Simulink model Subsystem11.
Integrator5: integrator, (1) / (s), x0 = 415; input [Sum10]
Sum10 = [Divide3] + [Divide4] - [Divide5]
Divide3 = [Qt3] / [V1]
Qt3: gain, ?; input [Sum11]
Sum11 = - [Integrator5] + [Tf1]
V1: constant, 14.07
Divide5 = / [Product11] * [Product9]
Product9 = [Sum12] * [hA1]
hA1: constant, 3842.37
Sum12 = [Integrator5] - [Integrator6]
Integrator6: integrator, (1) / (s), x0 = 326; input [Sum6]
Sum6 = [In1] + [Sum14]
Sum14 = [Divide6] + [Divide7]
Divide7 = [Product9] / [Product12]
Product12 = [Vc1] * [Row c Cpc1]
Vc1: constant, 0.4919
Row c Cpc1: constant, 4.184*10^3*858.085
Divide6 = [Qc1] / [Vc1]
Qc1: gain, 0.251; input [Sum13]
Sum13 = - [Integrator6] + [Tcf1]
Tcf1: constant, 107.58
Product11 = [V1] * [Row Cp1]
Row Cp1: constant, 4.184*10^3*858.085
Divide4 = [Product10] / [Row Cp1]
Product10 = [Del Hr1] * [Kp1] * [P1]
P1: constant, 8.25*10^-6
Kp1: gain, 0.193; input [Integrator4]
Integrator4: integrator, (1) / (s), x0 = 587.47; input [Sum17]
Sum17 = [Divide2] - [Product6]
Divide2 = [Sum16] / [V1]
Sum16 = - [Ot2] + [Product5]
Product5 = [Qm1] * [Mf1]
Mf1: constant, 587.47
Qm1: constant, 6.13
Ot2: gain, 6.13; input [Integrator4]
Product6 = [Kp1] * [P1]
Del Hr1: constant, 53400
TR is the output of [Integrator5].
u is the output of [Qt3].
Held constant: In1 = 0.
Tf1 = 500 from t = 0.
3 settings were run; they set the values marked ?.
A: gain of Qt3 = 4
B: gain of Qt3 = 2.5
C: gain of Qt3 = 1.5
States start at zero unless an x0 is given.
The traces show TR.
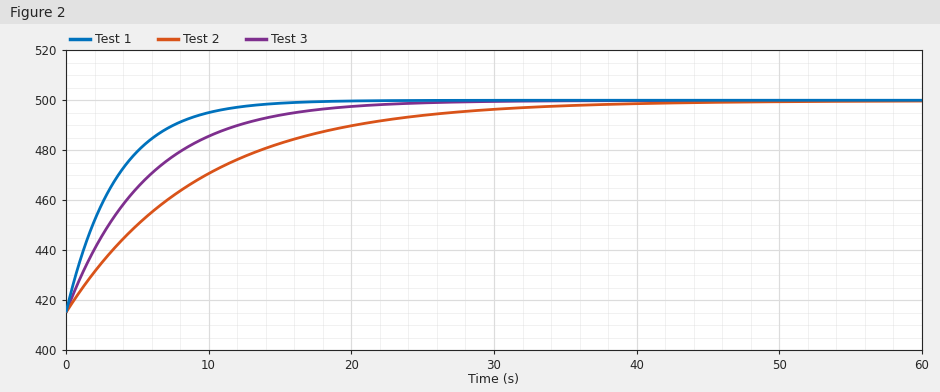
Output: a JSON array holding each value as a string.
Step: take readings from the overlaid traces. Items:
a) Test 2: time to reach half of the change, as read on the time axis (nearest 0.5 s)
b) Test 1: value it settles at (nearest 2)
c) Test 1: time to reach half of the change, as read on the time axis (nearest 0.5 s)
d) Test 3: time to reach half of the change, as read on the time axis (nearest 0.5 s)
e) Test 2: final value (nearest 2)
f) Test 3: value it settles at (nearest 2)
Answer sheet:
["6.5 s", "500", "2.5 s", "4.0 s", "500", "500"]
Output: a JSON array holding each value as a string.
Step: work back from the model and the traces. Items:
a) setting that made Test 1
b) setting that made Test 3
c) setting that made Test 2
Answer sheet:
["A", "B", "C"]
